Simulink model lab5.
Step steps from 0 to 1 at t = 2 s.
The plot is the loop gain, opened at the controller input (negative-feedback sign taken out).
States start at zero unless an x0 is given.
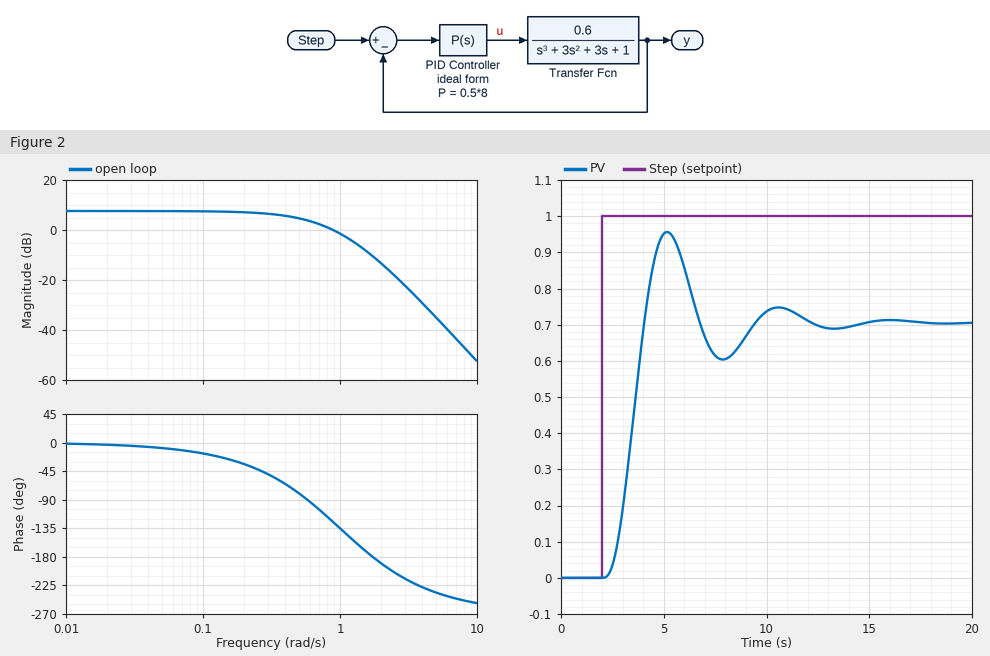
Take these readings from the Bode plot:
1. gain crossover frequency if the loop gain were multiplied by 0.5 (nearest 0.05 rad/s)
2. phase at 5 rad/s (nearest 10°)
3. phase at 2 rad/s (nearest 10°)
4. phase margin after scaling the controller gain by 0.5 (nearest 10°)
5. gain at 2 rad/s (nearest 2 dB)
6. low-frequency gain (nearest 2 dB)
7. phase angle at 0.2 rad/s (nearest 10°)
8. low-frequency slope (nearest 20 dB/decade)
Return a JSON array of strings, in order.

["0.35 rad/s", "-240°", "-190°", "120°", "-14 dB", "8 dB", "-30°", "0 dB/decade"]
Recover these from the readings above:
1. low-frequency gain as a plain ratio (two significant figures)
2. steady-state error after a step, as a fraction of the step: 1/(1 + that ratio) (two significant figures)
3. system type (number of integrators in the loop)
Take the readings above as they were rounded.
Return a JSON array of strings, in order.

["2.5", "0.29", "0"]
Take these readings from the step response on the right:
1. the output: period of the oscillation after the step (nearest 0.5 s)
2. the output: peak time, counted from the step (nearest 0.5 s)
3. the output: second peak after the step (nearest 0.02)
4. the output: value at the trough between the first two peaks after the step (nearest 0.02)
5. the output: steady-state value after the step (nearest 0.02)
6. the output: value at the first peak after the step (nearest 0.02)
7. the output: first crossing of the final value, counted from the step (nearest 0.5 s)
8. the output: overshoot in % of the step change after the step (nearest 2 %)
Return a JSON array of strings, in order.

["5.5 s", "3.0 s", "0.74", "0.60", "0.70", "0.96", "2.0 s", "36 %"]
